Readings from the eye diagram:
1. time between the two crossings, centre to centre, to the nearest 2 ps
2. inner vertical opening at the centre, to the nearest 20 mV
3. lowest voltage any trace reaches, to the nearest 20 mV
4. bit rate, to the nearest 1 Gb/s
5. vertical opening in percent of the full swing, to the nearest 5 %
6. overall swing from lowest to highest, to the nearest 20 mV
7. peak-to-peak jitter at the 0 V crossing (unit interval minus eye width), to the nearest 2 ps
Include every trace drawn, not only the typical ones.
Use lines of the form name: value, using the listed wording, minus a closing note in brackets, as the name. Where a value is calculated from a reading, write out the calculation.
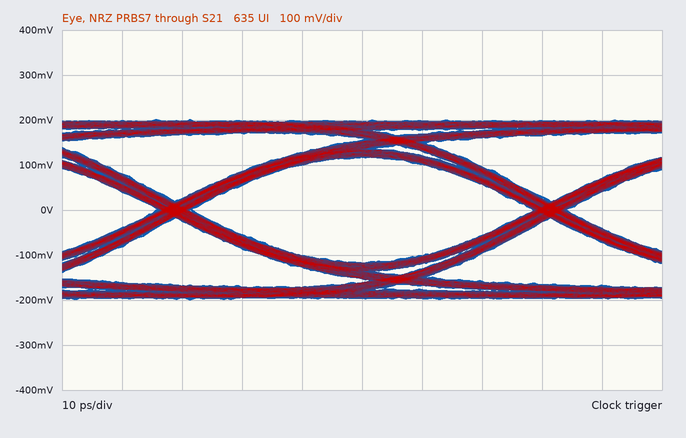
time between the two crossings, centre to centre, to the nearest 2 ps: 62 ps
inner vertical opening at the centre, to the nearest 20 mV: 240 mV
lowest voltage any trace reaches, to the nearest 20 mV: -200 mV
bit rate, to the nearest 1 Gb/s: 16 Gb/s
vertical opening in percent of the full swing, to the nearest 5 %: 240 mV / 400 mV ≈ 60 %
overall swing from lowest to highest, to the nearest 20 mV: 400 mV
peak-to-peak jitter at the 0 V crossing (unit interval minus eye width), to the nearest 2 ps: 6 ps
